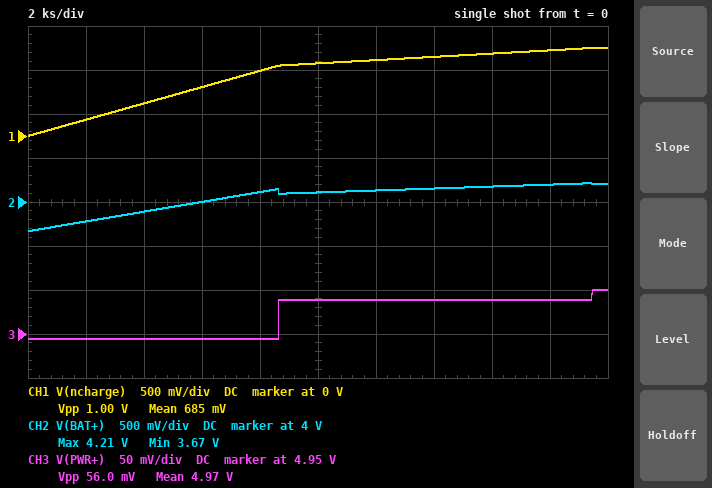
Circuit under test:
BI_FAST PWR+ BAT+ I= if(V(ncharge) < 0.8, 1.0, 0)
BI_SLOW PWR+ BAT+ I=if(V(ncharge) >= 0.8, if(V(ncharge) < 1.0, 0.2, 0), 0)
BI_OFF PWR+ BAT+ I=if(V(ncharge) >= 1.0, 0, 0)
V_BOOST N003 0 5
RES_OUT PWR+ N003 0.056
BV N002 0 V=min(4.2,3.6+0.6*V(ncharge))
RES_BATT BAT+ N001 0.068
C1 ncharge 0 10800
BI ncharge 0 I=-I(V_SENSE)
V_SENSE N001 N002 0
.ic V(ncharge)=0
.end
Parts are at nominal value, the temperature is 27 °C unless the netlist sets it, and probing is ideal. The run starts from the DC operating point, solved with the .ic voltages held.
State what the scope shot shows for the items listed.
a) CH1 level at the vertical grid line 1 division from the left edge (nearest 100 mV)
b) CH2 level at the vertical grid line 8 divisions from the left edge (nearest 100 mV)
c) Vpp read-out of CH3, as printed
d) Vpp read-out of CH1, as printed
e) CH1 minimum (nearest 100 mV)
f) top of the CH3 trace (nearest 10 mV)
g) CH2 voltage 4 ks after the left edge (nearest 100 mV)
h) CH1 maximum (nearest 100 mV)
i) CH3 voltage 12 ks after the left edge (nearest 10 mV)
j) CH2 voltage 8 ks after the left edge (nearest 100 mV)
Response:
200 mV
4.2 V
56.0 mV
1.00 V
0 V
5.00 V
3.9 V
1.0 V
4.99 V
4.1 V
